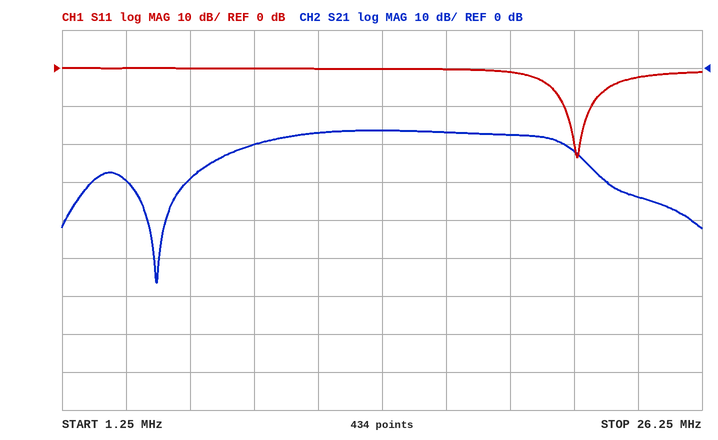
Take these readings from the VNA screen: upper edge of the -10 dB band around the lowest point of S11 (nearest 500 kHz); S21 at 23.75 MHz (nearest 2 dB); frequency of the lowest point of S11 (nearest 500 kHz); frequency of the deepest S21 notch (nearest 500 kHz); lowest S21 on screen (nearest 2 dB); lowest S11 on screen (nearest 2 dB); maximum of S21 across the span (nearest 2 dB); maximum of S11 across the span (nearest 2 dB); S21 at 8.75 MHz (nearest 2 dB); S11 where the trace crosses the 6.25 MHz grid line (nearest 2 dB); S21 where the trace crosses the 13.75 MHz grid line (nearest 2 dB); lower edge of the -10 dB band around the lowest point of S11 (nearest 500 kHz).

22.0 MHz
-34 dB
21.5 MHz
5.0 MHz
-56 dB
-24 dB
-16 dB
0 dB
-20 dB
0 dB
-16 dB
21.0 MHz
